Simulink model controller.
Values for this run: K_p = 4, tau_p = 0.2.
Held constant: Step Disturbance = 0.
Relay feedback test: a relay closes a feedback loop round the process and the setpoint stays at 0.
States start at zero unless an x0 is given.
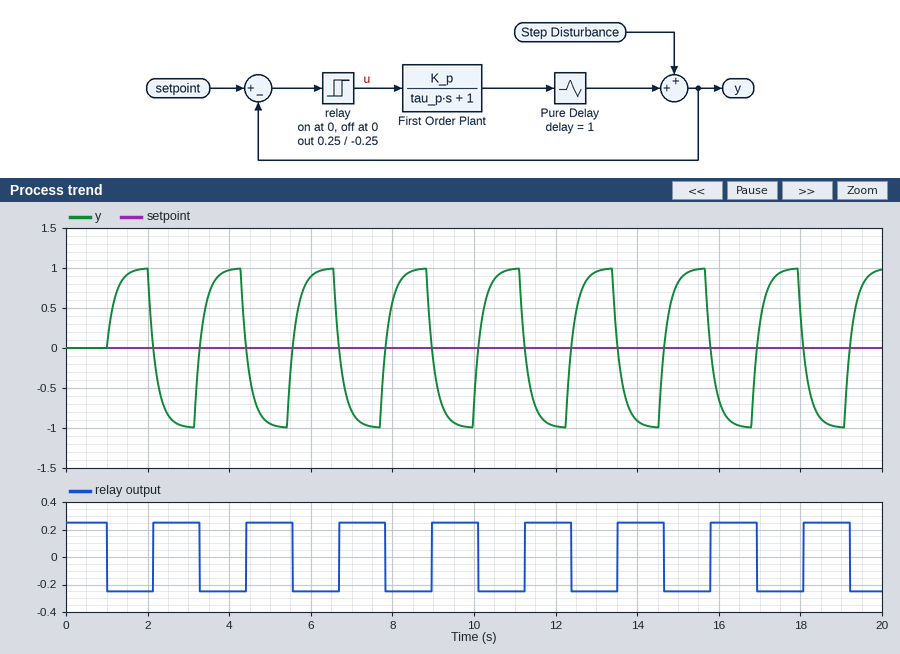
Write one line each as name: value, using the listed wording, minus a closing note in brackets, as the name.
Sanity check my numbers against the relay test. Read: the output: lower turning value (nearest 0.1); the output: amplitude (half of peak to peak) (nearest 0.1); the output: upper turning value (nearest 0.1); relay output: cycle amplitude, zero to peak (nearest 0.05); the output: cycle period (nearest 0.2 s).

the output: lower turning value: -1.0
the output: amplitude (half of peak to peak): 1.0
the output: upper turning value: 1.0
relay output: cycle amplitude, zero to peak: 0.25
the output: cycle period: 2.2 s
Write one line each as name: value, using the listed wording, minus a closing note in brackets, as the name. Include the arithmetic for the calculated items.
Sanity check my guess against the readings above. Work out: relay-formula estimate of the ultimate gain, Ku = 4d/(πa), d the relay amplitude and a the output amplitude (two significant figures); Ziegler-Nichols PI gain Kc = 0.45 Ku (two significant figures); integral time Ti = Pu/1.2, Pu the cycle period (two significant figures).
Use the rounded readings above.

relay-formula estimate of the ultimate gain, Ku = 4d/(πa), d the relay amplitude and a the output amplitude: 4 × 0.25 / (π × 1) = 0.32
Ziegler-Nichols PI gain Kc = 0.45 Ku: 0.45 × 0.32 = 0.14
integral time Ti = Pu/1.2, Pu the cycle period: 2.2 / 1.2 = 1.8 s
